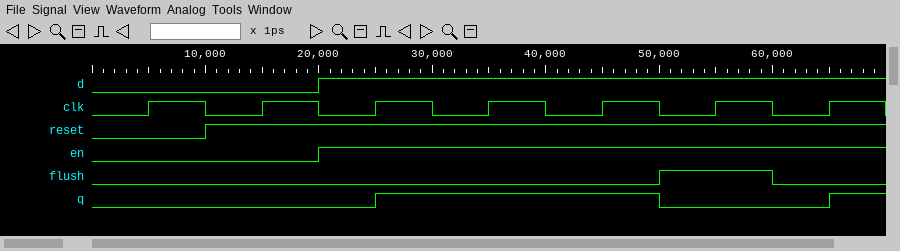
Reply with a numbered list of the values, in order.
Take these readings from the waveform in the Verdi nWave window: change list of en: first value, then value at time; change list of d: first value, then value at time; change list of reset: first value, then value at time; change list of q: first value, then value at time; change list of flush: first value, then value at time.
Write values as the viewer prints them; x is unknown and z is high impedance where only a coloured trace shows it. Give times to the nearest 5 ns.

1. 0, 1 at 20 ns
2. 0, 1 at 20 ns
3. 0, 1 at 10 ns
4. 0, 1 at 25 ns, 0 at 50 ns, 1 at 65 ns
5. 0, 1 at 50 ns, 0 at 60 ns
